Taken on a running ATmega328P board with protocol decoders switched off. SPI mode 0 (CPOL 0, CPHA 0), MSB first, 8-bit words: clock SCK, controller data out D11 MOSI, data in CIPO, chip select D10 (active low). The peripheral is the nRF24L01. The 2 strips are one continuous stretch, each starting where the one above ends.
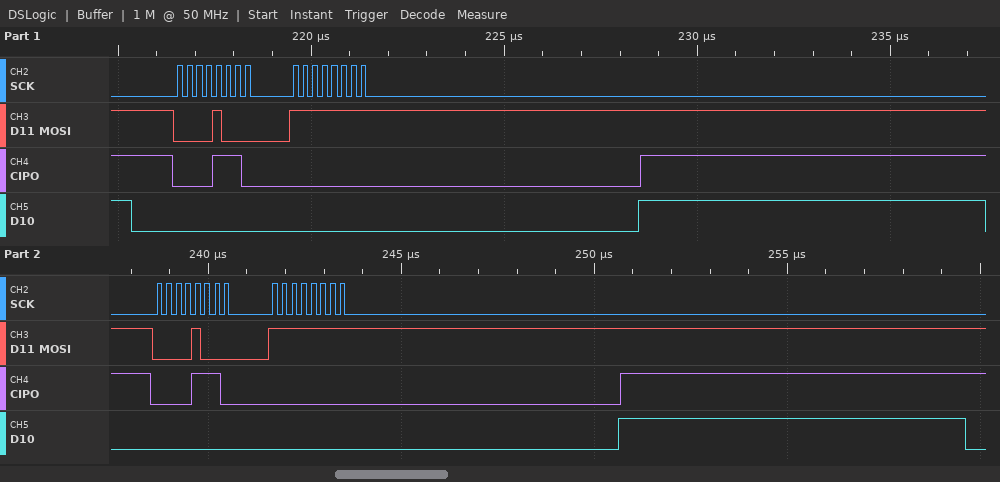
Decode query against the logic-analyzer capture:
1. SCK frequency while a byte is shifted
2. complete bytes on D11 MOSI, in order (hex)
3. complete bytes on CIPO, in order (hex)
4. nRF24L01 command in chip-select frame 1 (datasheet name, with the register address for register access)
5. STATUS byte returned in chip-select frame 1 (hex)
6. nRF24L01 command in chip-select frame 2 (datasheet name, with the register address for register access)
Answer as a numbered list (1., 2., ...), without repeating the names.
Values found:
1. 4 MHz
2. 0x08 0xFF 0x08 0xFF
3. 0x0E 0x00 0x0E 0x00
4. R_REGISTER 0x08
5. 0x0E
6. R_REGISTER 0x08
